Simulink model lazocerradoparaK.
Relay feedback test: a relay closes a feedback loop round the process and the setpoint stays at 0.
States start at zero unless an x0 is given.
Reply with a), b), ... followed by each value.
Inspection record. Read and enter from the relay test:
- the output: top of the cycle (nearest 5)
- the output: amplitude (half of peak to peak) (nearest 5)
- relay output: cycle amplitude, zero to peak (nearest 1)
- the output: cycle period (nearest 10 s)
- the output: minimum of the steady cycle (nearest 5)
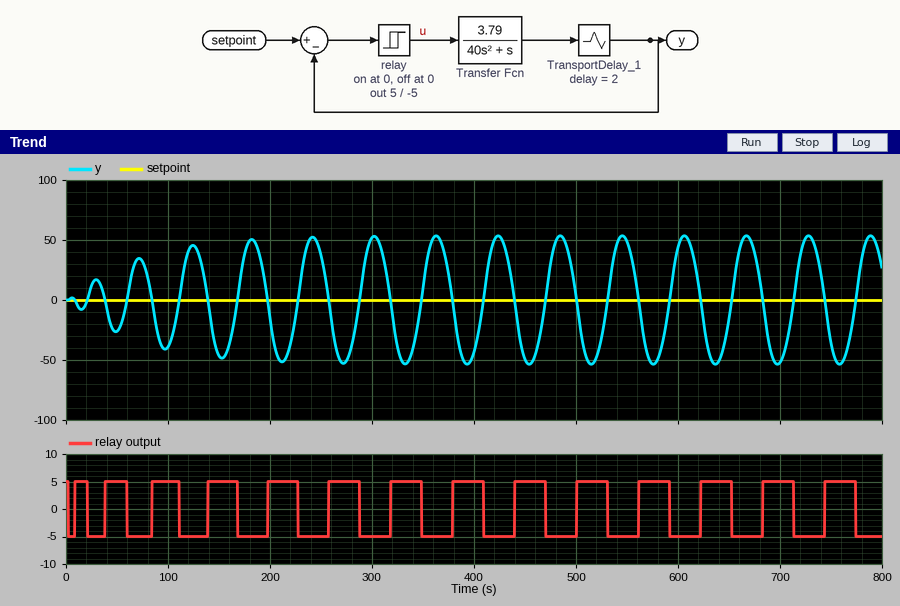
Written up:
a) 55
b) 55
c) 5
d) 60 s
e) -55
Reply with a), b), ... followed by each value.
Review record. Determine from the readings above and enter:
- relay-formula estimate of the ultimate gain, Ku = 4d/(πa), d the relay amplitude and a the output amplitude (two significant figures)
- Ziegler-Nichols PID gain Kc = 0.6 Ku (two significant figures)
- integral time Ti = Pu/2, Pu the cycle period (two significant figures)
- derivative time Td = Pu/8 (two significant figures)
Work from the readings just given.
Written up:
a) 0.12
b) 0.072
c) 30 s
d) 7.5 s
